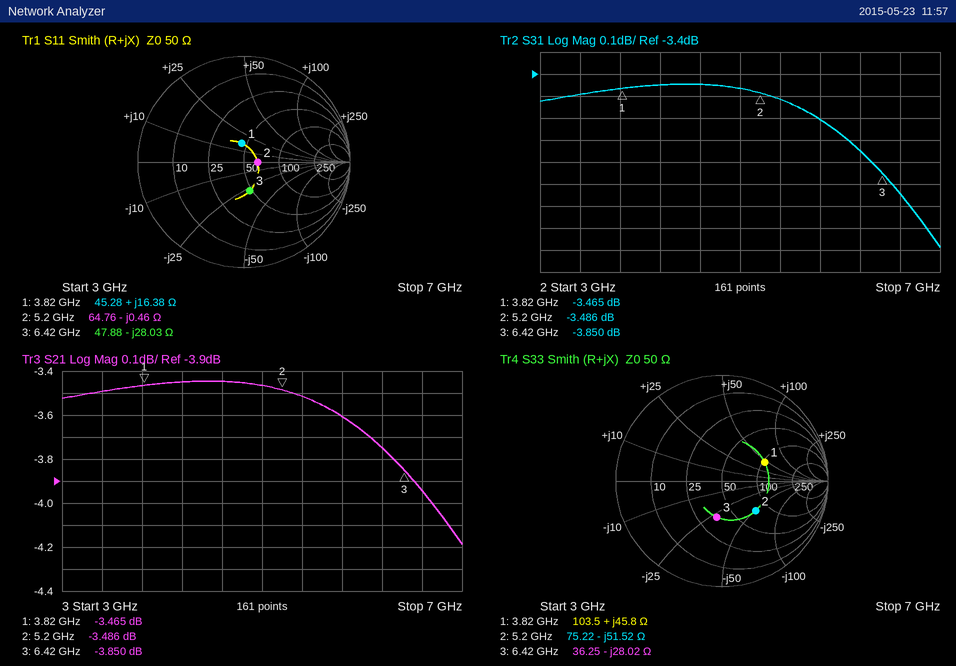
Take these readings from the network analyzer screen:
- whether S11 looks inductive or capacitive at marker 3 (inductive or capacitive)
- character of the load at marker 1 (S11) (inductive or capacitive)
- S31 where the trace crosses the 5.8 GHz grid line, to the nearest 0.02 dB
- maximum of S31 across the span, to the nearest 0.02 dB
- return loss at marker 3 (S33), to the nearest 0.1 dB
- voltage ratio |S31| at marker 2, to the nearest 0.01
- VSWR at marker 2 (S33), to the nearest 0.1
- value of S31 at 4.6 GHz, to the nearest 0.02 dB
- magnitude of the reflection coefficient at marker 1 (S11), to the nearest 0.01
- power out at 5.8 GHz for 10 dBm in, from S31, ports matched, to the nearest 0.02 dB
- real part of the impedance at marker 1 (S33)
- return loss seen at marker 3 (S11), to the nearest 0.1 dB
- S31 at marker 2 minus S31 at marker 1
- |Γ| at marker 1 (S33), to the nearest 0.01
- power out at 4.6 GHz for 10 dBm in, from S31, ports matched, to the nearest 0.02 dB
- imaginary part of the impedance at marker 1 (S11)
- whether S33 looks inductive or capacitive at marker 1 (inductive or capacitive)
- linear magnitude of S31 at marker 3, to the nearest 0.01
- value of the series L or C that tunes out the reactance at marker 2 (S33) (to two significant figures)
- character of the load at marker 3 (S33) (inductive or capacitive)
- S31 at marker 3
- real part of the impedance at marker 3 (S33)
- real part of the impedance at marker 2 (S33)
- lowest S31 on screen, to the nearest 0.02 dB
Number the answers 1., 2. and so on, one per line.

1. capacitive
2. inductive
3. -3.60 dB
4. -3.44 dB
5. 9.3 dB
6. 0.67
7. 2.5
8. -3.44 dB
9. 0.18
10. 6.40 dBm
11. 103.5 Ω
12. 11.2 dB
13. -0.021 dB
14. 0.44
15. 6.56 dBm
16. +16.38 Ω
17. inductive
18. 0.64
19. 1.6 nH
20. capacitive
21. -3.850 dB
22. 36.25 Ω
23. 75.22 Ω
24. -4.18 dB
